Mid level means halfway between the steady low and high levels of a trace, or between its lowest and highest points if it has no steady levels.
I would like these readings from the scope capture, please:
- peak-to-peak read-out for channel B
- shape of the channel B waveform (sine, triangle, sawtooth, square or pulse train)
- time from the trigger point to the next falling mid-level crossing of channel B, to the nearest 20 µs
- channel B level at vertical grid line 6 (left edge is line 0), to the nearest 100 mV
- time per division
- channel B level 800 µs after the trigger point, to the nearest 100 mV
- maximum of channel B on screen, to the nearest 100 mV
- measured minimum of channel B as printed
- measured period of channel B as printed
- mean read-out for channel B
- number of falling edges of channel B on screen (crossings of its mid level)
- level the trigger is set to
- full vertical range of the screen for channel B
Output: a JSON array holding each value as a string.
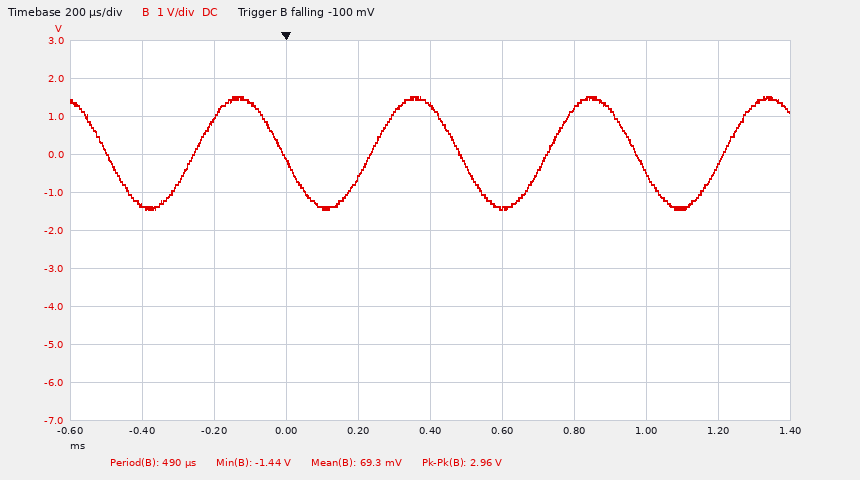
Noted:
["2.96 V", "sine", "480 µs", "-1.4 V", "200 µs", "1.2 V", "1.5 V", "-1.44 V", "490 µs", "69.3 mV", "4", "-100 mV", "10 V"]
